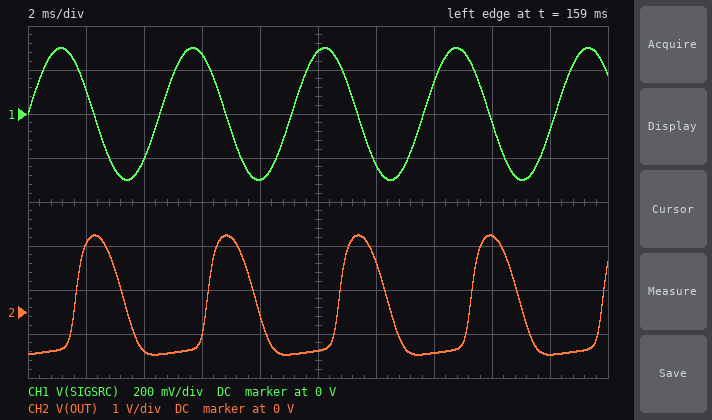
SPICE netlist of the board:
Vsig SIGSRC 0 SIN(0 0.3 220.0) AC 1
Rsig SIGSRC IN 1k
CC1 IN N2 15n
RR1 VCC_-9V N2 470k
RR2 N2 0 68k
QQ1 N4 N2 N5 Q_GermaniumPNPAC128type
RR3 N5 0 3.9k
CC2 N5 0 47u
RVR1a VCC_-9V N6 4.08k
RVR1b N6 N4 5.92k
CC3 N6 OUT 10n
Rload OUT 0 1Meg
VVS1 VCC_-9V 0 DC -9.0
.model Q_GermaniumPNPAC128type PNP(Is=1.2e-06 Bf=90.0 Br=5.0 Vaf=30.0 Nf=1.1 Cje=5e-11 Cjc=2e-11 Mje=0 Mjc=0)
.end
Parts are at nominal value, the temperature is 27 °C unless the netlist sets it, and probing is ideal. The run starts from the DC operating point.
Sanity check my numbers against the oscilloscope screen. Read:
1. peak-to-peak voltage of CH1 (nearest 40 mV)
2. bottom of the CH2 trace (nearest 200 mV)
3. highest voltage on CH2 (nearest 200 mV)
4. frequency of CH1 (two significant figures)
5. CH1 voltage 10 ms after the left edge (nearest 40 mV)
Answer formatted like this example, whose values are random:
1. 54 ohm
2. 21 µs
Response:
1. 600 mV
2. -1.0 V
3. 1.8 V
4. 220 Hz
5. 280 mV
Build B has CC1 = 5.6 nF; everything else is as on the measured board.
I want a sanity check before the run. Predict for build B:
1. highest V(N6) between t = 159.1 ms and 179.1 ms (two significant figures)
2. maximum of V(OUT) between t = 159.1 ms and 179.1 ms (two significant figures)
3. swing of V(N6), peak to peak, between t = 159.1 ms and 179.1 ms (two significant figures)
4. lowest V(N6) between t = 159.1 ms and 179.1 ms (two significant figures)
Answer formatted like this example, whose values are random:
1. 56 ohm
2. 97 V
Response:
1. -7.3 V
2. 750 mV
3. 1.4 V
4. -8.8 V
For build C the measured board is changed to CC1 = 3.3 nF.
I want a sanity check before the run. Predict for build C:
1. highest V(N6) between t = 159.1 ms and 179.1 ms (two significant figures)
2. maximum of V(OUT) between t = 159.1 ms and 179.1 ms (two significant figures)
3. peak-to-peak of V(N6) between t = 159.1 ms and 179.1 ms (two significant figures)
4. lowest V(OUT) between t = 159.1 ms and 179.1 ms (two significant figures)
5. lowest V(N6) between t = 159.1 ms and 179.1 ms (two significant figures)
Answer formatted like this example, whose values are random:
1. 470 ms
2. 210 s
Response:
1. -7.6 V
2. 450 mV
3. 890 mV
4. -440 mV
5. -8.5 V
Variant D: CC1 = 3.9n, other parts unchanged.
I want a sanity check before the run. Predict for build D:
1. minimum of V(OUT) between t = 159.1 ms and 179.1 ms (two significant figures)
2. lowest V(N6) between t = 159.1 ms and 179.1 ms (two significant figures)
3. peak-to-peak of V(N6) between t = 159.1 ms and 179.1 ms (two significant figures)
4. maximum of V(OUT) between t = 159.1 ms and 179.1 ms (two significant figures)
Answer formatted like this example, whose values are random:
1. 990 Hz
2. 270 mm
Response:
1. -510 mV
2. -8.6 V
3. 1.0 V
4. 530 mV
